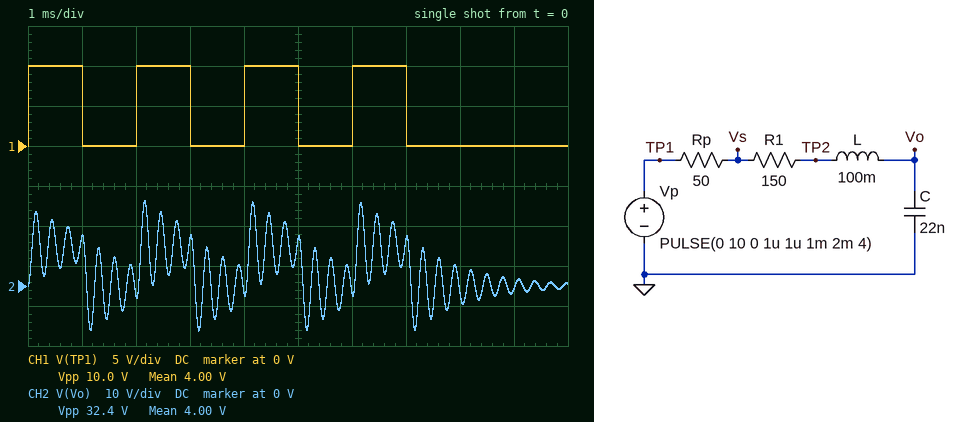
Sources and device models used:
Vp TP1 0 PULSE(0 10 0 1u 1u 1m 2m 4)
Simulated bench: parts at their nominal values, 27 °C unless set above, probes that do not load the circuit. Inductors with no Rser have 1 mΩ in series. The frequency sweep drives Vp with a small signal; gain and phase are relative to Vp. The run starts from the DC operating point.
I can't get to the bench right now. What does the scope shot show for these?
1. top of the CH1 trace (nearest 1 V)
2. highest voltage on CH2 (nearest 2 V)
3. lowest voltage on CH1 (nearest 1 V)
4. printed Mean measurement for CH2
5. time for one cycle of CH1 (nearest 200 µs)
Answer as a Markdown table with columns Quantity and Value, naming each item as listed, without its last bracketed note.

| Quantity | Value |
|---|---|
| top of the CH1 trace | 10 V |
| highest voltage on CH2 | 22 V |
| lowest voltage on CH1 | 0 V |
| printed Mean measurement for CH2 | 4.00 V |
| time for one cycle of CH1 | 2.0 ms |
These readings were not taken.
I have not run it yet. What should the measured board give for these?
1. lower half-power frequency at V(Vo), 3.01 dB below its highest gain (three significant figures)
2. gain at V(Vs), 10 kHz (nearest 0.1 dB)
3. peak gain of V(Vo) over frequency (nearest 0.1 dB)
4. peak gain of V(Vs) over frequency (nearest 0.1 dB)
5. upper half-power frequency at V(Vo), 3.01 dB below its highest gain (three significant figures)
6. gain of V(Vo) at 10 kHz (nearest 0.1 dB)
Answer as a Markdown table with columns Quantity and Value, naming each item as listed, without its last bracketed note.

| Quantity | Value |
|---|---|
| lower half-power frequency at V(Vo), 3.01 dB below its highest gain | 3.22 kHz |
| gain at V(Vs), 10 kHz | 0 dB |
| peak gain of V(Vo) over frequency | 20.6 dB |
| peak gain of V(Vs) over frequency | 0 dB |
| upper half-power frequency at V(Vo), 3.01 dB below its highest gain | 3.54 kHz |
| gain of V(Vo) at 10 kHz | -17.7 dB |
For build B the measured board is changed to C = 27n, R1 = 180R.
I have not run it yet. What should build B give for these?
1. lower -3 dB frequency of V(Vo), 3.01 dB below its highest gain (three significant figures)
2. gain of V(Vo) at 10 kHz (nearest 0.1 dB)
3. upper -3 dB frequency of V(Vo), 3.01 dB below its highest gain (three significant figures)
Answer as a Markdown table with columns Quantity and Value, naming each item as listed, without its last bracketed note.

| Quantity | Value |
|---|---|
| lower -3 dB frequency of V(Vo), 3.01 dB below its highest gain | 2.86 kHz |
| gain of V(Vo) at 10 kHz | -19.7 dB |
| upper -3 dB frequency of V(Vo), 3.01 dB below its highest gain | 3.23 kHz |
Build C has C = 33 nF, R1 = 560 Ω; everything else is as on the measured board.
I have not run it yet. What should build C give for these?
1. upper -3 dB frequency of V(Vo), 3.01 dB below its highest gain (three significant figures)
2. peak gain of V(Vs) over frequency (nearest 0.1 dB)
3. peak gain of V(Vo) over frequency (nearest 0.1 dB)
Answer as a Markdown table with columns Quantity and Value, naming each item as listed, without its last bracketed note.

| Quantity | Value |
|---|---|
| upper -3 dB frequency of V(Vo), 3.01 dB below its highest gain | 3.14 kHz |
| peak gain of V(Vs) over frequency | 0 dB |
| peak gain of V(Vo) over frequency | 9.2 dB |
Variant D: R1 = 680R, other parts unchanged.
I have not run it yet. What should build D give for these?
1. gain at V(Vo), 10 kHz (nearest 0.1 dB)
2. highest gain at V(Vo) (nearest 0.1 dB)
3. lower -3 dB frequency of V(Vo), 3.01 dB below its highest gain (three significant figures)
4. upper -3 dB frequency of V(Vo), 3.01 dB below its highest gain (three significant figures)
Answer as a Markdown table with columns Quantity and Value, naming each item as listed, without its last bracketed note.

| Quantity | Value |
|---|---|
| gain at V(Vo), 10 kHz | -17.8 dB |
| highest gain at V(Vo) | 9.4 dB |
| lower -3 dB frequency of V(Vo), 3.01 dB below its highest gain | 2.64 kHz |
| upper -3 dB frequency of V(Vo), 3.01 dB below its highest gain | 3.84 kHz |
